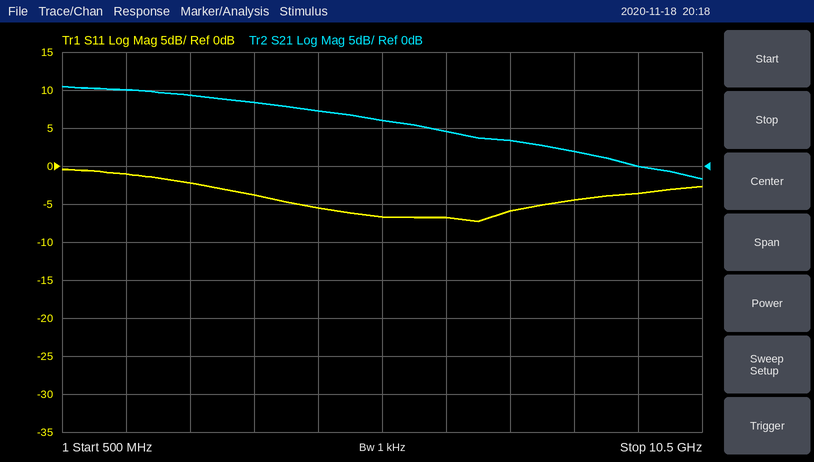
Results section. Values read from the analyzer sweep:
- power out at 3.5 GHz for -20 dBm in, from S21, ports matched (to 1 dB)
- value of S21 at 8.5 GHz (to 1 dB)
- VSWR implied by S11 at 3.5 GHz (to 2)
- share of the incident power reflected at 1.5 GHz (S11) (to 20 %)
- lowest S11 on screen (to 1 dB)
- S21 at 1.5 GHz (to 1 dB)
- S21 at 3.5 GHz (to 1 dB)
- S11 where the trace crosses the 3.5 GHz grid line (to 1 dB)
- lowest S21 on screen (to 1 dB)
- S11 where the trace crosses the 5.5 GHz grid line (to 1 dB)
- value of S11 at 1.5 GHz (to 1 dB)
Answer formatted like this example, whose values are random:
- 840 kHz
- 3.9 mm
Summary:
- -12 dBm
- 2 dB
- 4
- 80 %
- -7 dB
- 10 dB
- 8 dB
- -4 dB
- -2 dB
- -7 dB
- -1 dB
